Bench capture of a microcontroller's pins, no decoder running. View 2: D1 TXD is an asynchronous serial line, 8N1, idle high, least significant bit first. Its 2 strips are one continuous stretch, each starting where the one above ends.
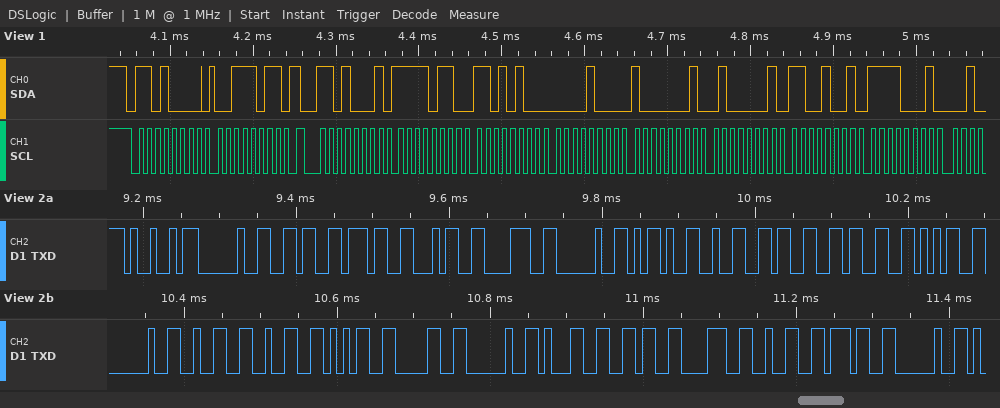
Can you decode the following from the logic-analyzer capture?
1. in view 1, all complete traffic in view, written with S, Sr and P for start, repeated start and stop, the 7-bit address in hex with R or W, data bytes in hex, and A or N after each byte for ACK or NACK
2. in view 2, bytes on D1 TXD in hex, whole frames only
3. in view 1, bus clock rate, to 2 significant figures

S 68W A 3B A Sr 68R A F6 A D4 A 08 A 81 A 41 A C9 A F1 A
49 20 36 37 34 38 20 2D 32 33 33 35 20 32 32 35 30 20 31 36 38 32 37 20
100 kHz
